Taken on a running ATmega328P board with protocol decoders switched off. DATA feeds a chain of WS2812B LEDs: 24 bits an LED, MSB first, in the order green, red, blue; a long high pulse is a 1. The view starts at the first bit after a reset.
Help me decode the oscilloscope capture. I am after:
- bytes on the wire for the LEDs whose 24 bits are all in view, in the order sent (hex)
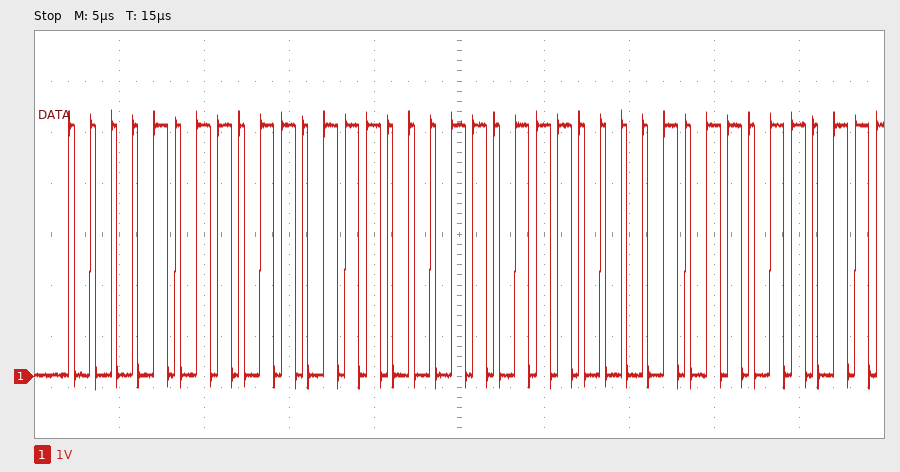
0B 6E 37
